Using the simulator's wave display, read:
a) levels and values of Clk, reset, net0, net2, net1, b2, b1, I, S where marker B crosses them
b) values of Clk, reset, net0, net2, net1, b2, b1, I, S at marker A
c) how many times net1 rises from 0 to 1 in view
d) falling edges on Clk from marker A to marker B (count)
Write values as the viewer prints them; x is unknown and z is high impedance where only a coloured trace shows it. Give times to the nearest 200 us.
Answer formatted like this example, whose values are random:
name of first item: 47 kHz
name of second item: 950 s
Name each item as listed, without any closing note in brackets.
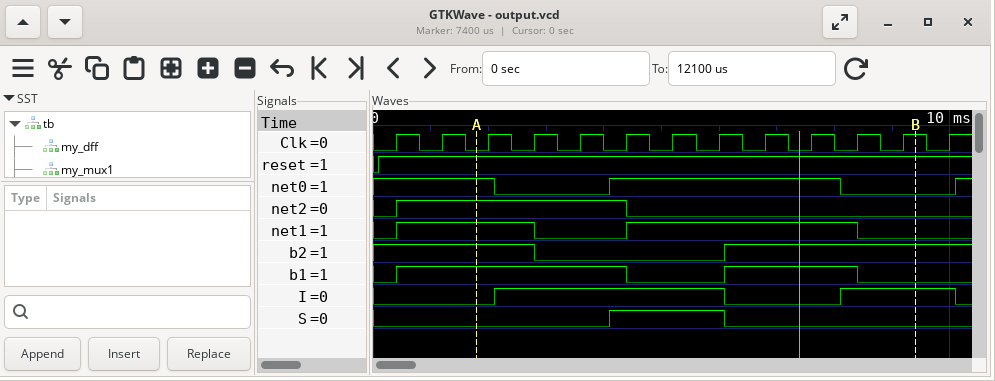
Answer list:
levels and values of Clk, reset, net0, net2, net1, b2, b1, I, S where marker B crosses them: Clk=1, reset=1, net0=0, net2=0, net1=0, b2=1, b1=0, I=1, S=0
values of Clk, reset, net0, net2, net1, b2, b1, I, S at marker A: Clk=0, reset=1, net0=1, net2=1, net1=1, b2=1, b1=1, I=0, S=0
how many times net1 rises from 0 to 1 in view: 2
falling edges on Clk from marker A to marker B: 9
